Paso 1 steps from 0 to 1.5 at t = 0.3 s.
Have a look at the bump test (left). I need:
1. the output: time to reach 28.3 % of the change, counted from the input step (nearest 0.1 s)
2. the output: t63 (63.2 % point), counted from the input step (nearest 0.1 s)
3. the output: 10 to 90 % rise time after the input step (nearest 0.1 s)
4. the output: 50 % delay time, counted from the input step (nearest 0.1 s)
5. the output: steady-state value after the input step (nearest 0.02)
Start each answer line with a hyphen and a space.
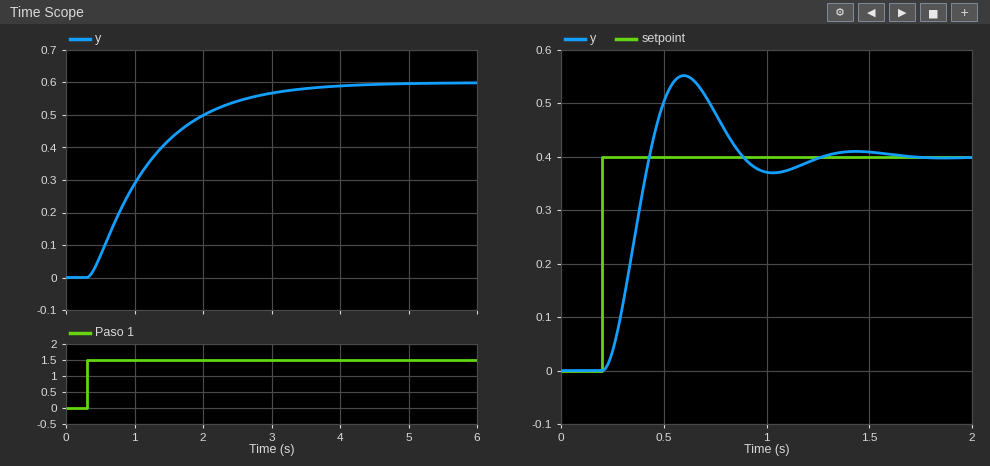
- 0.4 s
- 1.0 s
- 2.0 s
- 0.7 s
- 0.60
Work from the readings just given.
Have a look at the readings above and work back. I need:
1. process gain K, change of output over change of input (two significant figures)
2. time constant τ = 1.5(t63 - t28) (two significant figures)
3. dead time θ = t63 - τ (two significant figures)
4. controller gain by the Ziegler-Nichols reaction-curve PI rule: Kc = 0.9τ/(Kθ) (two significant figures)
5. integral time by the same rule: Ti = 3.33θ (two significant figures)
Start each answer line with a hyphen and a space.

- 0.40
- 0.90 s
- 0.10 s
- 20
- 0.33 s
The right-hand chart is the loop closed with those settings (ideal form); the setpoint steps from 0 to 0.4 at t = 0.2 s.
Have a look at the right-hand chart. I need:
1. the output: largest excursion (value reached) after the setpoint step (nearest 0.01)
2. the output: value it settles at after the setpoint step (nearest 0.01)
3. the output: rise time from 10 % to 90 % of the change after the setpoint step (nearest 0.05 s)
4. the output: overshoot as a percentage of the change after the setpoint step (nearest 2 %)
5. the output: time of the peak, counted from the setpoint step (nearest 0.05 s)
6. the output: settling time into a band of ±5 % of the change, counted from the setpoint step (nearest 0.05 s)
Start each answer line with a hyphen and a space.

- 0.55
- 0.40
- 0.15 s
- 38 %
- 0.40 s
- 0.95 s
